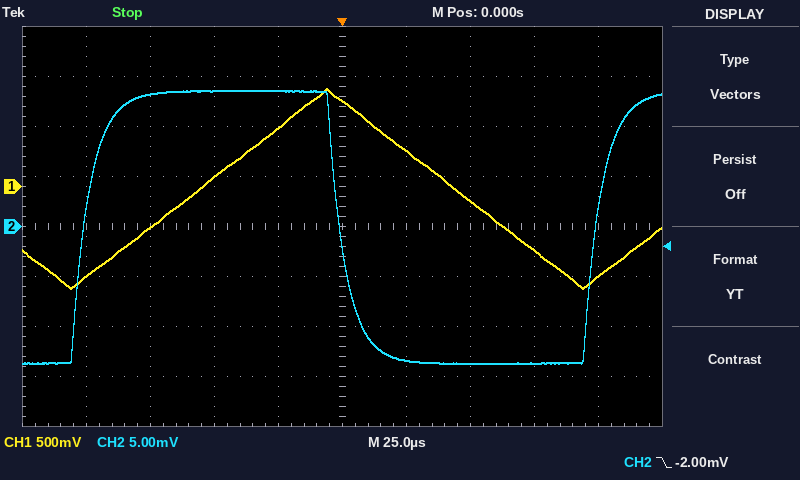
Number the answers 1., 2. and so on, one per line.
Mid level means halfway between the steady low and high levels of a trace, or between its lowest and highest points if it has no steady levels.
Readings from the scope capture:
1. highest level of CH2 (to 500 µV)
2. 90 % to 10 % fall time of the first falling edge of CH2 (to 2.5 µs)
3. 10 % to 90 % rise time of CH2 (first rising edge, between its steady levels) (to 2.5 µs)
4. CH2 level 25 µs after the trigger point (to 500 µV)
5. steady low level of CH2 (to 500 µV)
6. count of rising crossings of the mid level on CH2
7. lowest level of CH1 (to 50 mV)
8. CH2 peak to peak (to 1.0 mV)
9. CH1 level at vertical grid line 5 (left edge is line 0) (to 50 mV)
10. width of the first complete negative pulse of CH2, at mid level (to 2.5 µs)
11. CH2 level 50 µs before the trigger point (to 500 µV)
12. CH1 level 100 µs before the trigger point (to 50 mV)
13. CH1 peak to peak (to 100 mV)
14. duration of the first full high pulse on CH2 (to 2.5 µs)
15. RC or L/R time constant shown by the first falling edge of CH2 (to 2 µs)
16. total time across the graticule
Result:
1. 13.5 mV
2. 15.0 µs
3. 15.0 µs
4. -13.5 mV
5. -13.5 mV
6. 2
7. -1.00 V
8. 27.0 mV
9. 850 mV
10. 100.0 µs
11. 13.5 mV
12. -900 mV
13. 2.00 V
14. 100.0 µs
15. 6 µs
16. 250 µs
